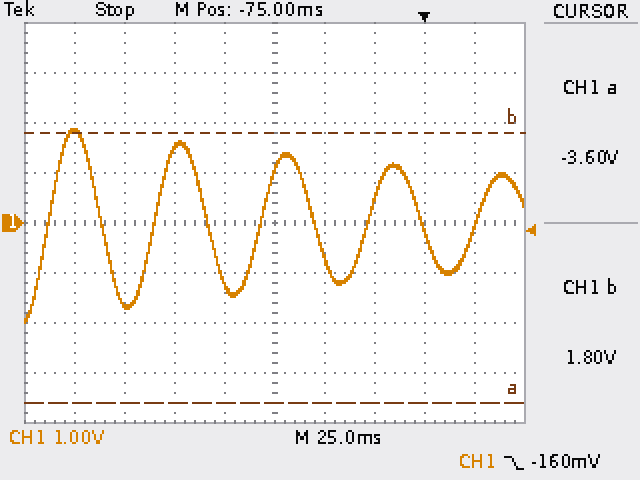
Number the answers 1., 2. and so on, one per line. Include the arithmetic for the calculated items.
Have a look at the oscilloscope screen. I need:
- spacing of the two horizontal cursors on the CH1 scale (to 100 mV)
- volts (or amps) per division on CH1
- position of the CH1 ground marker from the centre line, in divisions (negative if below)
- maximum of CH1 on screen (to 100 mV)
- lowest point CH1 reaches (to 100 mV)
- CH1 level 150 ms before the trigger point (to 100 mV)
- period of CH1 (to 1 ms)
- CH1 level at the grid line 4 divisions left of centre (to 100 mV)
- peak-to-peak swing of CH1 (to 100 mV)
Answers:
1. 5.4 V
2. 1 V
3. 0.0 div
4. 1.9 V
5. -2.0 V
6. -1.6 V
7. 53 ms
8. 1.8 V
9. 1.9 V − (-2.0 V) = 3.9 V
